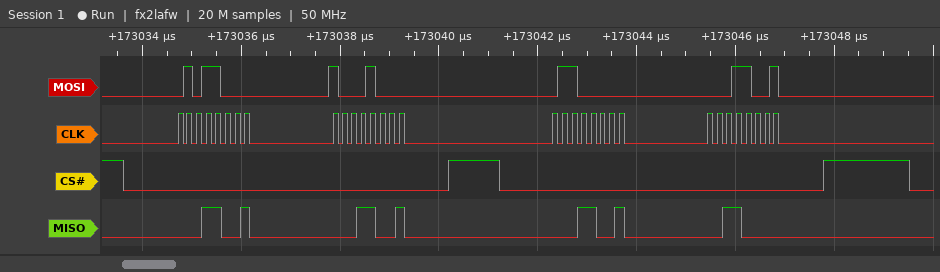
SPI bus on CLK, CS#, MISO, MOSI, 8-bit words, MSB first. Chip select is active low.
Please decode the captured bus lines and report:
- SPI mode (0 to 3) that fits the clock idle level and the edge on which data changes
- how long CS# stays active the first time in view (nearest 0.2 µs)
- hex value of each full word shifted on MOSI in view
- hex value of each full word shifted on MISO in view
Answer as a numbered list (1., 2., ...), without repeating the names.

1. 0
2. 6.6 µs
3. 58, 88, 60, 19
4. 19, 19, 19, 30
